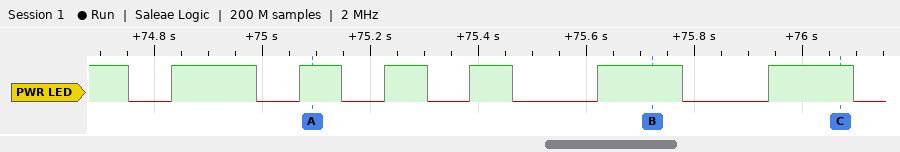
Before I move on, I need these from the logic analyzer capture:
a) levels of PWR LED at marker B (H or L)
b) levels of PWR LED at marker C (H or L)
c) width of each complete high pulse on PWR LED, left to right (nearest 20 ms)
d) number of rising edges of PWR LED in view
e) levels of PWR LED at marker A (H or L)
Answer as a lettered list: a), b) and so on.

a) PWR LED=H
b) PWR LED=H
c) 160 ms, 80 ms, 80 ms, 80 ms, 160 ms, 160 ms
d) 6
e) PWR LED=H
